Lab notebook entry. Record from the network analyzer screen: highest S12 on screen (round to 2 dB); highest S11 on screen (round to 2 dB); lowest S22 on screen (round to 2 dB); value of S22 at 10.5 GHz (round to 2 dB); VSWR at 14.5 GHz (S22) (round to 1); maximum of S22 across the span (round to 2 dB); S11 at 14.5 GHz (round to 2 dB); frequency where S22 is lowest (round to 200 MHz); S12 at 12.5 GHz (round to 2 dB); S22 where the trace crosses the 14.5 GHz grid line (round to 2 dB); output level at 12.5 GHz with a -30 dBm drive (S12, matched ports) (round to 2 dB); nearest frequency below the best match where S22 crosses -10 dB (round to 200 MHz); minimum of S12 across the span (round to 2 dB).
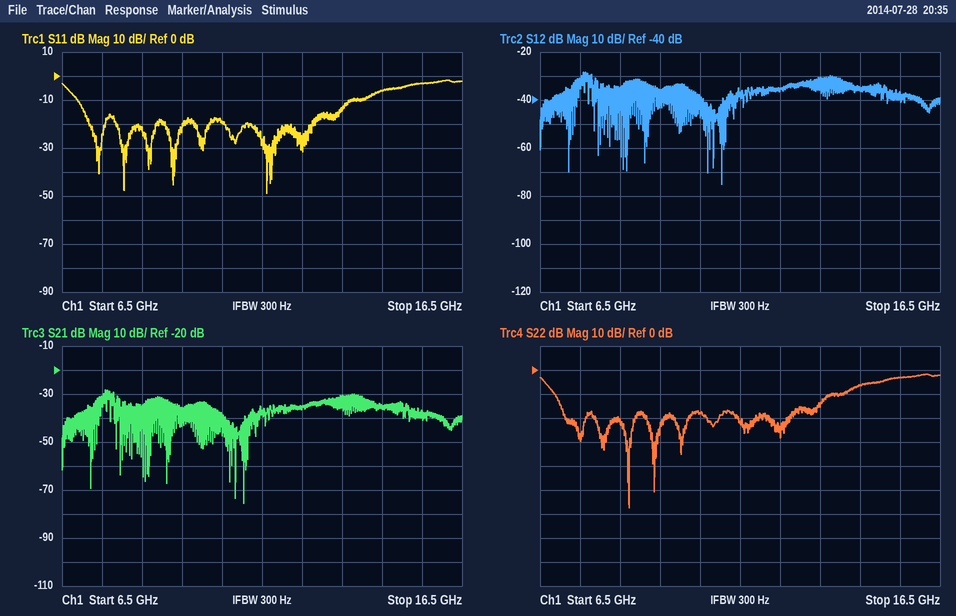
-28 dB
-2 dB
-58 dB
-18 dB
3
-2 dB
-6 dB
8.8 GHz
-36 dB
-6 dB
-66 dBm
6.8 GHz
-76 dB
